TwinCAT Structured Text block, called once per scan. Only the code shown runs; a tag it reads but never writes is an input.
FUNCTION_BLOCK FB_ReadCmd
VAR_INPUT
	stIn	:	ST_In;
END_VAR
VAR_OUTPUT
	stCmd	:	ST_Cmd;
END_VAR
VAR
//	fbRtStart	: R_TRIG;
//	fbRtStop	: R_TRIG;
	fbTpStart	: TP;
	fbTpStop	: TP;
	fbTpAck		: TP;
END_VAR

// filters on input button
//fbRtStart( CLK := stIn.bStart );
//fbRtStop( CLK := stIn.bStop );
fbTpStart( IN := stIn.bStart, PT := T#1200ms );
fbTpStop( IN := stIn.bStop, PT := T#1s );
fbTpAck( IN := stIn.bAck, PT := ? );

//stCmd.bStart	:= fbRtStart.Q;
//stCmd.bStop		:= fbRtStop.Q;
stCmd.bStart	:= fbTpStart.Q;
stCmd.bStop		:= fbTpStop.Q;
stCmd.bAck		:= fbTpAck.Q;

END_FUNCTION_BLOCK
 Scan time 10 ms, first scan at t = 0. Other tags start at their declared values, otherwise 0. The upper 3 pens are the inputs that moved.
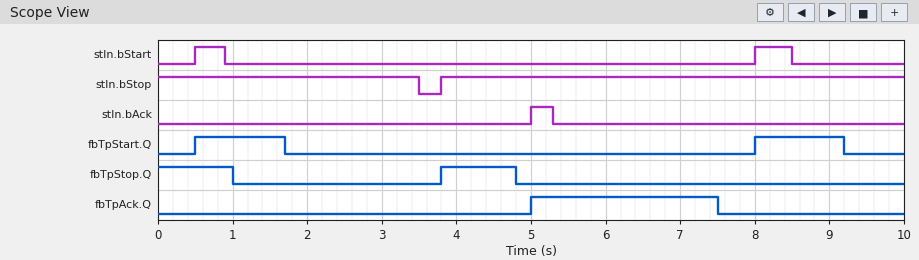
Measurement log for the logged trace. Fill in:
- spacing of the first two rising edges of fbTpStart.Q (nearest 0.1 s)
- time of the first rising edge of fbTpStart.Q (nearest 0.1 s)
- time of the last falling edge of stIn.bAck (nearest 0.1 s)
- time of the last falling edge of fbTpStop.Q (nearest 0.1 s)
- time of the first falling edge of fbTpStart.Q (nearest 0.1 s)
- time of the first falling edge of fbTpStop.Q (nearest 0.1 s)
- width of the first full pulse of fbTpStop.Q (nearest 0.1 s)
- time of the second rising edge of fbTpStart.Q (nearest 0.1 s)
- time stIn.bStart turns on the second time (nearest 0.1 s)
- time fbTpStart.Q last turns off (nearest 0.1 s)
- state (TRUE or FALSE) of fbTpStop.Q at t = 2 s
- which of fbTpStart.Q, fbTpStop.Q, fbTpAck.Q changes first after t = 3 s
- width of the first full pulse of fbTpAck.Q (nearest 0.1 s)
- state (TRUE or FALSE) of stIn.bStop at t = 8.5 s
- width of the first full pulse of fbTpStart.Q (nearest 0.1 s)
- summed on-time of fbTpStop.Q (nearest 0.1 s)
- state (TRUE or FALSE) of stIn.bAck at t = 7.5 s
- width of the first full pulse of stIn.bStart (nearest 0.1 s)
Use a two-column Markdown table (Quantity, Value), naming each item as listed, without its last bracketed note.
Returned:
| Quantity | Value |
|---|---|
| spacing of the first two rising edges of fbTpStart.Q | 7.5 s |
| time of the first rising edge of fbTpStart.Q | 0.5 s |
| time of the last falling edge of stIn.bAck | 5.3 s |
| time of the last falling edge of fbTpStop.Q | 4.8 s |
| time of the first falling edge of fbTpStart.Q | 1.7 s |
| time of the first falling edge of fbTpStop.Q | 1.0 s |
| width of the first full pulse of fbTpStop.Q | 1.0 s |
| time of the second rising edge of fbTpStart.Q | 8.0 s |
| time stIn.bStart turns on the second time | 8.0 s |
| time fbTpStart.Q last turns off | 9.2 s |
| state (TRUE or FALSE) of fbTpStop.Q at t = 2 s | FALSE |
| which of fbTpStart.Q, fbTpStop.Q, fbTpAck.Q changes first after t = 3 s | fbTpStop.Q |
| width of the first full pulse of fbTpAck.Q | 2.5 s |
| state (TRUE or FALSE) of stIn.bStop at t = 8.5 s | TRUE |
| width of the first full pulse of fbTpStart.Q | 1.2 s |
| summed on-time of fbTpStop.Q | 2.0 s |
| state (TRUE or FALSE) of stIn.bAck at t = 7.5 s | FALSE |
| width of the first full pulse of stIn.bStart | 0.4 s |
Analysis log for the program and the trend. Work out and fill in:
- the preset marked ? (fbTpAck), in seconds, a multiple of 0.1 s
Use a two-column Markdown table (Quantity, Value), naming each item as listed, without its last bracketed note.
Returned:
| Quantity | Value |
|---|---|
| the preset marked ? (fbTpAck), in seconds, a multiple of 0.1 s | 2.5 s |
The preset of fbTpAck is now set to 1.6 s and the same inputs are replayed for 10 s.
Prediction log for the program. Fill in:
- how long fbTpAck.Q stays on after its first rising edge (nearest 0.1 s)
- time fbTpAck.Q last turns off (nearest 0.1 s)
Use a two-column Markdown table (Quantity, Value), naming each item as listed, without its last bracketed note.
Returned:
| Quantity | Value |
|---|---|
| how long fbTpAck.Q stays on after its first rising edge | 1.6 s |
| time fbTpAck.Q last turns off | 6.6 s |
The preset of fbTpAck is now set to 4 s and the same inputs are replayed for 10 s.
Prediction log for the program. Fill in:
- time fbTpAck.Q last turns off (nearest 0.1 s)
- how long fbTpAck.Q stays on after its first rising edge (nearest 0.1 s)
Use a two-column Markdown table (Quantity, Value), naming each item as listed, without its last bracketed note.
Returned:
| Quantity | Value |
|---|---|
| time fbTpAck.Q last turns off | 9.0 s |
| how long fbTpAck.Q stays on after its first rising edge | 4.0 s |
